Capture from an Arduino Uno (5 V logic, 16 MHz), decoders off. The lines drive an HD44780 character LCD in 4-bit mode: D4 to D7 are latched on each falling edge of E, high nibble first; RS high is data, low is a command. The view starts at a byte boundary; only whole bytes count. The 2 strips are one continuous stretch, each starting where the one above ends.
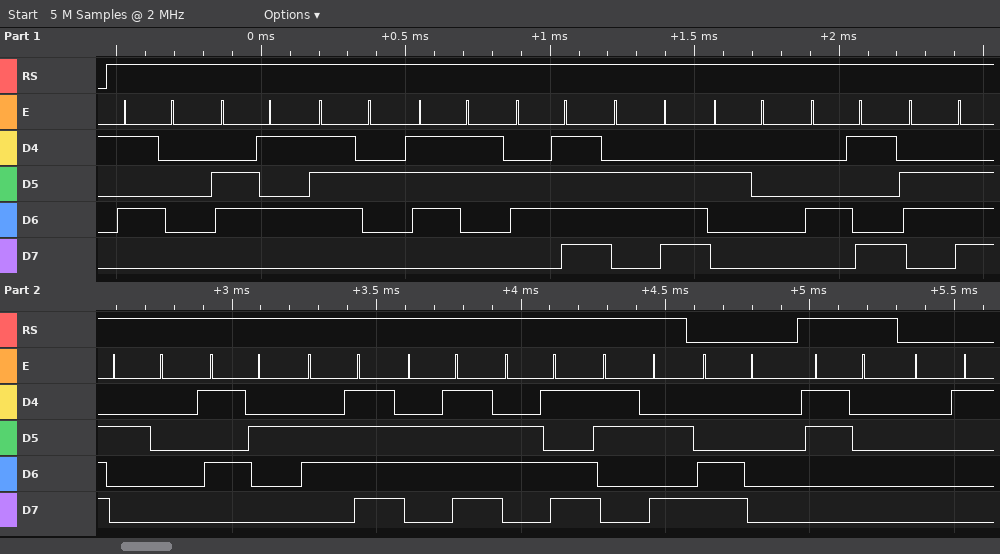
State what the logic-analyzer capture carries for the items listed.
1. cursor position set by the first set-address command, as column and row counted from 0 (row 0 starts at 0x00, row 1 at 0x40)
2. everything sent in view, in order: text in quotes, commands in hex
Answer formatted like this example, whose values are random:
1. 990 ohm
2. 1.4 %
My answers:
1. column 0, row 1
2. "Person In Room:" 0xC0 "0" 0x01
